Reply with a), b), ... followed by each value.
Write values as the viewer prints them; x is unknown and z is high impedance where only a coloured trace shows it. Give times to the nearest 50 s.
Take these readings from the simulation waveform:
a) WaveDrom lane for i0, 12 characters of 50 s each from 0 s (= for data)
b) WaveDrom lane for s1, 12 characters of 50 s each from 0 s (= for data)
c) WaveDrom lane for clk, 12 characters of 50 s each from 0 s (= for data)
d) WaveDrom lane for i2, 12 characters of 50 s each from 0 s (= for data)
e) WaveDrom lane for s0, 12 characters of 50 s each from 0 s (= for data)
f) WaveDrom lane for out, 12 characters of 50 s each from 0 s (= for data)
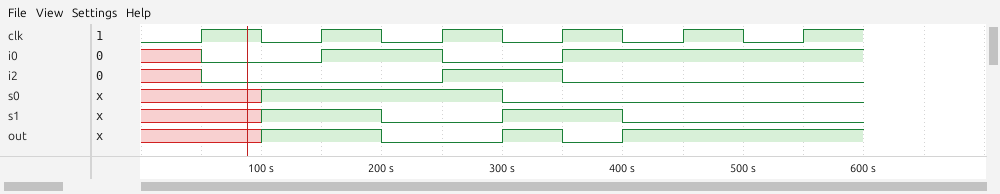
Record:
a) {name: 'i0', wave: 'x0.1.0.1....'}
b) {name: 's1', wave: 'x.1.0.1.0...'}
c) {name: 'clk', wave: '010101010101'}
d) {name: 'i2', wave: 'x0...1.0....'}
e) {name: 's0', wave: 'x.1...0.....'}
f) {name: 'out', wave: 'x.1.0.101...'}
